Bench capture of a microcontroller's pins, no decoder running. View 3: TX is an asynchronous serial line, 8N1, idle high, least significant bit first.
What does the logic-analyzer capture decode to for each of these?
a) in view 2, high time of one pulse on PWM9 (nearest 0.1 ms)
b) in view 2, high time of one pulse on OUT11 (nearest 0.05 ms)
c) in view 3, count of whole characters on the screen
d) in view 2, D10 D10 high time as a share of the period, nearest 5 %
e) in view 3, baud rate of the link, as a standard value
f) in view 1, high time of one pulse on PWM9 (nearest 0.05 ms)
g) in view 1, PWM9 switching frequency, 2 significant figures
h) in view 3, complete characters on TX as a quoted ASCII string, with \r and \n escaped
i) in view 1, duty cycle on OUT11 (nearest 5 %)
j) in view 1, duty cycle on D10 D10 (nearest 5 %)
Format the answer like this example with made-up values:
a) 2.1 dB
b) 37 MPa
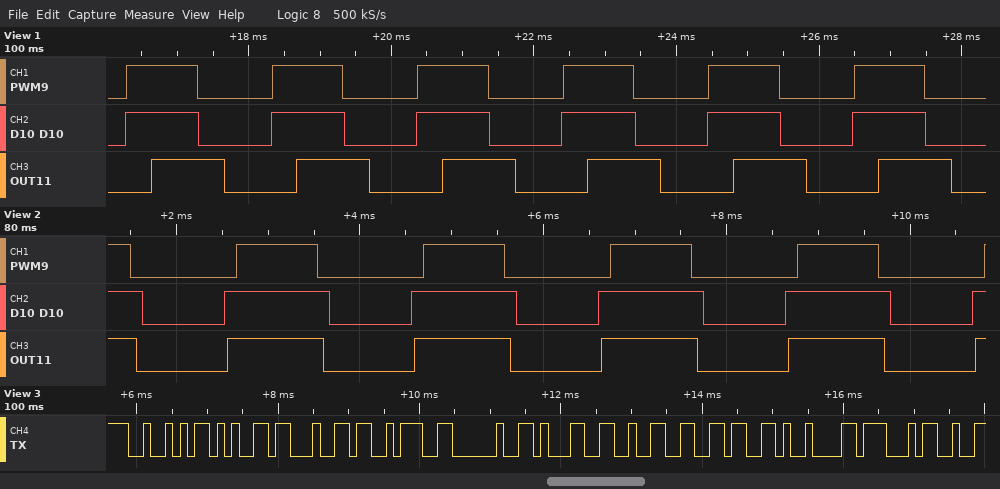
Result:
a) 0.9 ms
b) 1.05 ms
c) 10
d) 55 %
e) 9600 baud
f) 1.00 ms
g) 490 Hz
h) "Red: 126\tG"
i) 50 %
j) 50 %
